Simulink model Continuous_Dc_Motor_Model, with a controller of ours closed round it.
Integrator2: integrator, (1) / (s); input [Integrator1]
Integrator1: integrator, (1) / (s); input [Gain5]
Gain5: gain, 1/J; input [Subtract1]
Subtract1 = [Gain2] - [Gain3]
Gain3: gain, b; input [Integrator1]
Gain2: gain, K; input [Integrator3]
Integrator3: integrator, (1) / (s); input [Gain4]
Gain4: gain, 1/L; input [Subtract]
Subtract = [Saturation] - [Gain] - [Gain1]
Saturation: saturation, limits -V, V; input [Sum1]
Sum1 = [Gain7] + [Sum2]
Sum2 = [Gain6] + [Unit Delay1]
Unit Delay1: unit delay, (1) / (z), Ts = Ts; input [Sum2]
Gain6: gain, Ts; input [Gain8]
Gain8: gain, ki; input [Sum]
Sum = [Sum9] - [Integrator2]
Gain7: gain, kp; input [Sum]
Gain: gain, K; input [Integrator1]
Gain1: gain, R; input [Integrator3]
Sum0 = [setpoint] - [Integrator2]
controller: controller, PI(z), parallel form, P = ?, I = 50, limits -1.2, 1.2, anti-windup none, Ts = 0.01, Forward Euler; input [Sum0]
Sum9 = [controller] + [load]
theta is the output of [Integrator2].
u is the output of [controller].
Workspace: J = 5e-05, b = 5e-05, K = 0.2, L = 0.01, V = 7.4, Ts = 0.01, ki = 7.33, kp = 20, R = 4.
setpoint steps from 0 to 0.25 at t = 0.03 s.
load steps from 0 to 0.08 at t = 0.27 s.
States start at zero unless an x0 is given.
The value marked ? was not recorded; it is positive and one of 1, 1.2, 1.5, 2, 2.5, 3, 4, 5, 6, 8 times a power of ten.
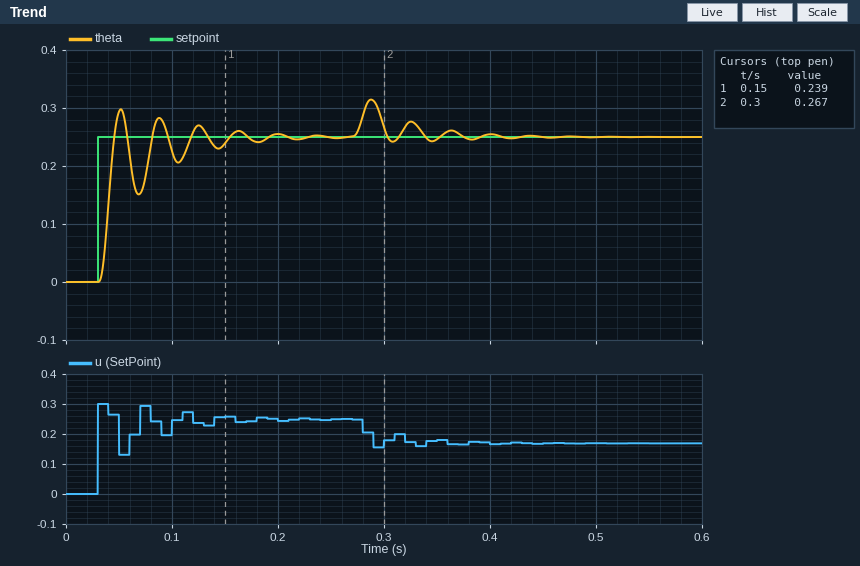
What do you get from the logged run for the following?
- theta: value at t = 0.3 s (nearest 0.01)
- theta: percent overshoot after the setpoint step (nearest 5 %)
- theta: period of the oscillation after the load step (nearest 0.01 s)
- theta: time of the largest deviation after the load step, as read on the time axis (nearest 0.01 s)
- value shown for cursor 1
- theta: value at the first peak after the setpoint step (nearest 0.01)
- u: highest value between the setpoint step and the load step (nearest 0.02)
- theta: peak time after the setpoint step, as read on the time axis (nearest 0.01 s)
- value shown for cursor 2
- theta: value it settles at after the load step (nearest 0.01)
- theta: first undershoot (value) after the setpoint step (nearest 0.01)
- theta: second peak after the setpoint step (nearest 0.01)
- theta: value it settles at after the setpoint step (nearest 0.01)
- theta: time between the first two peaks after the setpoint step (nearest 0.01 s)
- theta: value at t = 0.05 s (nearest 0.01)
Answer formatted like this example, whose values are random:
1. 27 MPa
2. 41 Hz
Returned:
1. 0.27
2. 20 %
3. 0.04 s
4. 0.29 s
5. 0.239
6. 0.30
7. 0.30
8. 0.05 s
9. 0.267
10. 0.25
11. 0.15
12. 0.28
13. 0.25
14. 0.04 s
15. 0.29
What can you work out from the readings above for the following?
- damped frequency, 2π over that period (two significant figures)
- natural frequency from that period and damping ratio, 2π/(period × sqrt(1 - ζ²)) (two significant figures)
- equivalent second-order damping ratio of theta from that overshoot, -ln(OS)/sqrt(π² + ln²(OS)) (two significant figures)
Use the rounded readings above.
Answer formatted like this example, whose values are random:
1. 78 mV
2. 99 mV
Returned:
1. 160 rad/s
2. 180 rad/s
3. 0.46
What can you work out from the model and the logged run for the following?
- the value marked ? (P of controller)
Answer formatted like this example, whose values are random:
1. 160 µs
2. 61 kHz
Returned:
1. 1.2
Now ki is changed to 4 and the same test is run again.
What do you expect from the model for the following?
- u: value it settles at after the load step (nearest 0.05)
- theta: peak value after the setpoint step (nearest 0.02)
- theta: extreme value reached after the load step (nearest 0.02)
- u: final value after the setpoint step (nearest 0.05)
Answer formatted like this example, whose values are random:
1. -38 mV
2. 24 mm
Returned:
1. 0.15
2. 0.30
3. 0.32
4. 0.25
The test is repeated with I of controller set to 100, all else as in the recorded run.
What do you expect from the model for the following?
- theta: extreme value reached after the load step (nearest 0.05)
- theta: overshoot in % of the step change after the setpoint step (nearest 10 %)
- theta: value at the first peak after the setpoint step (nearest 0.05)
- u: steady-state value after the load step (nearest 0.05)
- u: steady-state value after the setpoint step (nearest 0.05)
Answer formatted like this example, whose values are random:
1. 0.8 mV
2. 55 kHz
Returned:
1. 0.30
2. 50 %
3. 0.40
4. 0.15
5. 0.25
